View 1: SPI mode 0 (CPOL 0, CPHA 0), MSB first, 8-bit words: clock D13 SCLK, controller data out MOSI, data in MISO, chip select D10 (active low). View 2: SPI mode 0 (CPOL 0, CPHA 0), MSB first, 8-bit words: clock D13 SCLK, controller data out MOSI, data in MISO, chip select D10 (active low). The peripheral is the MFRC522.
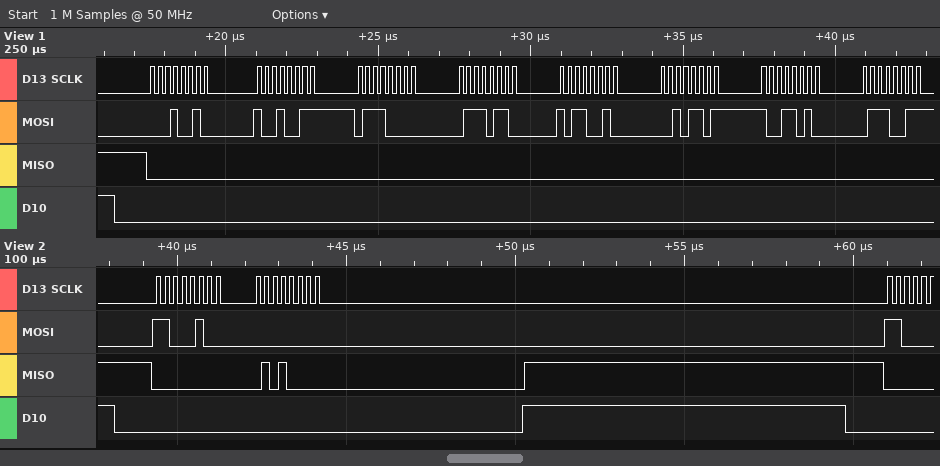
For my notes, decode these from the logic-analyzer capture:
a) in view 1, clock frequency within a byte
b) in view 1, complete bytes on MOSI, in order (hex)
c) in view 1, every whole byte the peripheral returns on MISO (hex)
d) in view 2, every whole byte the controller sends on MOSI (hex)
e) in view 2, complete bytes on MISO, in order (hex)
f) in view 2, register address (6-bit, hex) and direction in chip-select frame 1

4 MHz
0x12 0x93 0x70 0x76 0xB2 0x2D 0x9A 0x73
0x00 0x00 0x00 0x00 0x00 0x00 0x00 0x00
C4 00
00 50
0x22 read
